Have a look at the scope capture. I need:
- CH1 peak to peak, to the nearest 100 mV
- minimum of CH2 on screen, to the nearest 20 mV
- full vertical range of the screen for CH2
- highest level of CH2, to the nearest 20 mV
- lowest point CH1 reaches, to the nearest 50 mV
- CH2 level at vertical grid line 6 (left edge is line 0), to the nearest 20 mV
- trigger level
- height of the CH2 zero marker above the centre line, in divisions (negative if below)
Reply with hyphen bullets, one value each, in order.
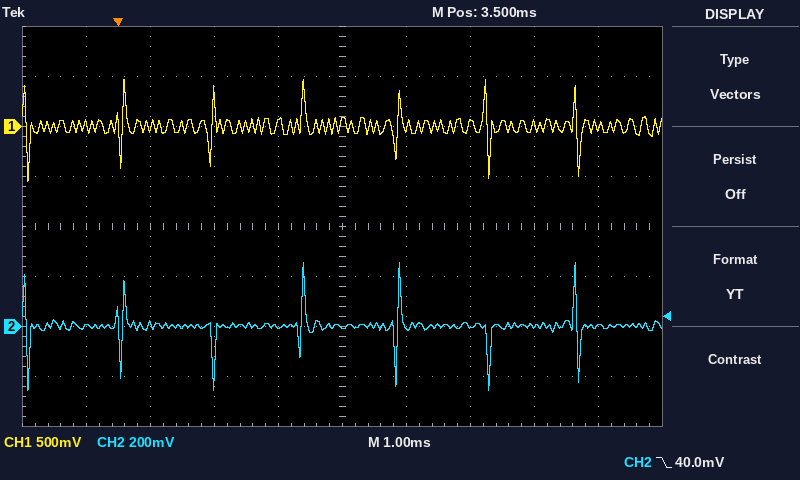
- 1.00 V
- -260 mV
- 1.6 V
- 260 mV
- -550 mV
- 0 mV
- 40.0 mV
- -2.0 div
